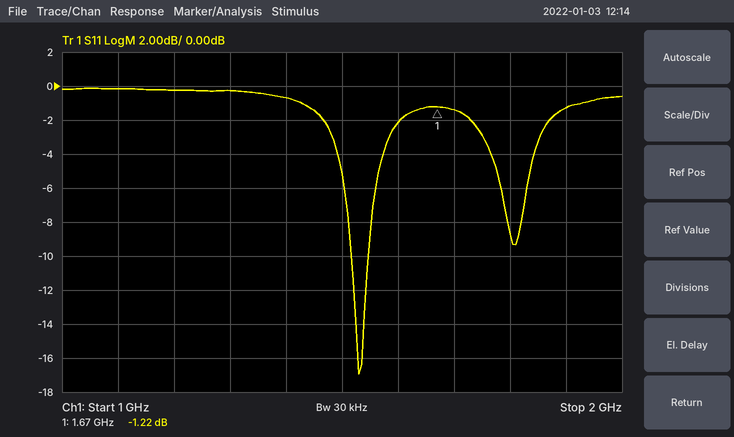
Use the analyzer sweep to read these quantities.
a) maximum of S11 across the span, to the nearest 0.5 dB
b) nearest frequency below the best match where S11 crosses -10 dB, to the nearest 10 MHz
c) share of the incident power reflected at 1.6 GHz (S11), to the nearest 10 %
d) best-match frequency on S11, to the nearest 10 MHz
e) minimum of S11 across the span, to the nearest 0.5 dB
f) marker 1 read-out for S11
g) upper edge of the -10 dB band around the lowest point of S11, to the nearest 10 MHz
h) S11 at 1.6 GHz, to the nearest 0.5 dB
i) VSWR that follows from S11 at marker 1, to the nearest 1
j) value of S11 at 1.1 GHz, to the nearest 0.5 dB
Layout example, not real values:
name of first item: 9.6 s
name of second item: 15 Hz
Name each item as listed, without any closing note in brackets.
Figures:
maximum of S11 across the span, to the nearest 0.5 dB: 0.0 dB
nearest frequency below the best match where S11 crosses -10 dB, to the nearest 10 MHz: 1.52 GHz
share of the incident power reflected at 1.6 GHz (S11), to the nearest 10 %: 60 %
best-match frequency on S11, to the nearest 10 MHz: 1.53 GHz
minimum of S11 across the span, to the nearest 0.5 dB: -17.0 dB
marker 1 read-out for S11: -1.22 dB
upper edge of the -10 dB band around the lowest point of S11, to the nearest 10 MHz: 1.55 GHz
S11 at 1.6 GHz, to the nearest 0.5 dB: -2.0 dB
VSWR that follows from S11 at marker 1, to the nearest 1: 14
value of S11 at 1.1 GHz, to the nearest 0.5 dB: 0.0 dB
